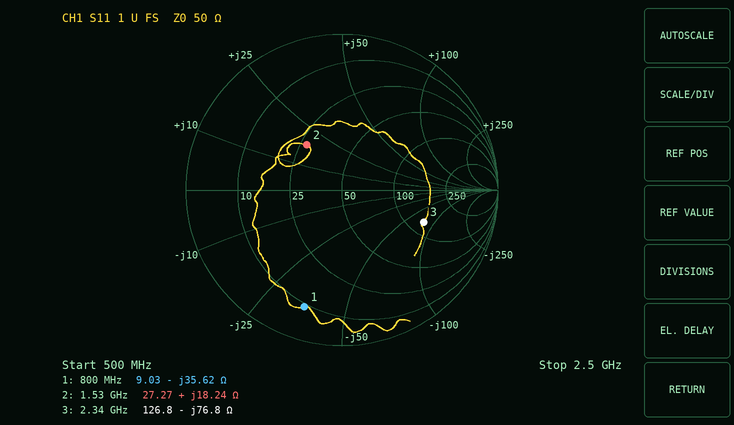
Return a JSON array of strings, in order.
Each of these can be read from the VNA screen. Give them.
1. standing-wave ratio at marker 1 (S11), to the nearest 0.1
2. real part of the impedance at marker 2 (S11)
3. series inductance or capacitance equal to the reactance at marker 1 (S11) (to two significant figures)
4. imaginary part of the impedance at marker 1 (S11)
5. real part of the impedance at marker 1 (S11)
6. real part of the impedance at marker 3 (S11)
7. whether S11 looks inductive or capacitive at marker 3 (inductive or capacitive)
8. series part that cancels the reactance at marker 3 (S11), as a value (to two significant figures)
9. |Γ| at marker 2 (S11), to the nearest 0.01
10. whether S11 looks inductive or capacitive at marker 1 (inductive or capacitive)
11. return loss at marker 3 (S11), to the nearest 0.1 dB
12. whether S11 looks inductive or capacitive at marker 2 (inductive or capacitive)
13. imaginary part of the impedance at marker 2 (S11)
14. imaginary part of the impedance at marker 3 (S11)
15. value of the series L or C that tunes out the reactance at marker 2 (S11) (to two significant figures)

["8.4", "27.27 Ω", "5.6 pF", "-35.62 Ω", "9.03 Ω", "126.8 Ω", "capacitive", "5.2 nH", "0.37", "capacitive", "5.0 dB", "inductive", "+18.24 Ω", "-76.8 Ω", "5.7 pF"]
